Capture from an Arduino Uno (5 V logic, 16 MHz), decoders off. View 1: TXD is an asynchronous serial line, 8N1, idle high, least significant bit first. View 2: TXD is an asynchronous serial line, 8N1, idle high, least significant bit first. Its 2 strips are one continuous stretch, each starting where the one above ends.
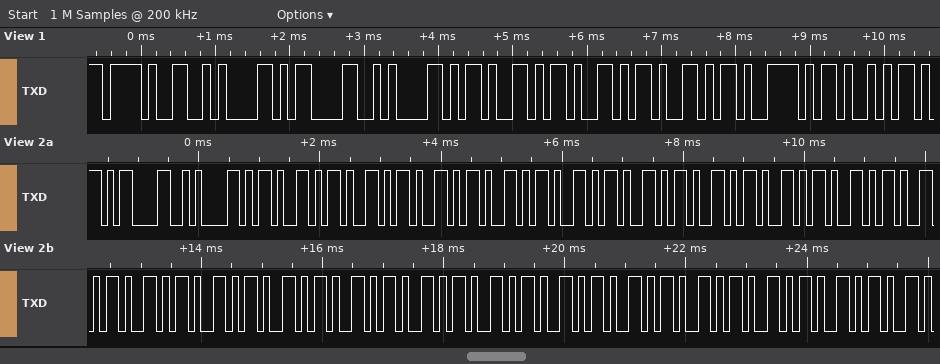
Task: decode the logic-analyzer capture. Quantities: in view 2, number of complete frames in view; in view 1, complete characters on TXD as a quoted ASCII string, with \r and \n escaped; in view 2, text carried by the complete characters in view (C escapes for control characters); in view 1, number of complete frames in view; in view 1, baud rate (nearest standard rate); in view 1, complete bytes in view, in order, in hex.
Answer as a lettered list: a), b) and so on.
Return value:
a) 24
b) "/\n\r\n-----"
c) "\r\n----------------------"
d) 9
e) 9600 baud
f) 2F 0A 0D 0A 2D 2D 2D 2D 2D
